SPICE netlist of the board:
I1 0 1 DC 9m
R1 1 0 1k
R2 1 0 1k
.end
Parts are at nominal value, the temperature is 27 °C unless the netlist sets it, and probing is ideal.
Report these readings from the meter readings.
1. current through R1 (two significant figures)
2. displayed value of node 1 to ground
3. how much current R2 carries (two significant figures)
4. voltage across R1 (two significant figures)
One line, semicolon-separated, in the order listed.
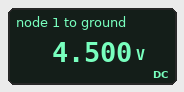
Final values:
4.5 mA; 4.500 V; 4.5 mA; 4.5 V
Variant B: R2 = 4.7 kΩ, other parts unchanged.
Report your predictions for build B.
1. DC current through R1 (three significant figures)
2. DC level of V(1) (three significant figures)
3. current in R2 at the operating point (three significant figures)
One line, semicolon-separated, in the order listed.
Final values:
7.42 mA; 7.42 V; 1.58 mA
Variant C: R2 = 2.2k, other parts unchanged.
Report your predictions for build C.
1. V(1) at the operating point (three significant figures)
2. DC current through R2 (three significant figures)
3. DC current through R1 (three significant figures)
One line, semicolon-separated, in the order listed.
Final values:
6.19 V; 2.81 mA; 6.19 mA
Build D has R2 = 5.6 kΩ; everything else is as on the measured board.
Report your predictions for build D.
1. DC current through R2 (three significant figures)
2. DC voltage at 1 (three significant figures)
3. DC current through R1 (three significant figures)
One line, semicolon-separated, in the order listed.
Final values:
1.36 mA; 7.64 V; 7.64 mA
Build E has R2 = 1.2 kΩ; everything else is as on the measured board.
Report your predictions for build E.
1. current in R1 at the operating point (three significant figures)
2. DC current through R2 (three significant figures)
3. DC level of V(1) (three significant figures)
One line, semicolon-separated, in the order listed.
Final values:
4.91 mA; 4.09 mA; 4.91 V
